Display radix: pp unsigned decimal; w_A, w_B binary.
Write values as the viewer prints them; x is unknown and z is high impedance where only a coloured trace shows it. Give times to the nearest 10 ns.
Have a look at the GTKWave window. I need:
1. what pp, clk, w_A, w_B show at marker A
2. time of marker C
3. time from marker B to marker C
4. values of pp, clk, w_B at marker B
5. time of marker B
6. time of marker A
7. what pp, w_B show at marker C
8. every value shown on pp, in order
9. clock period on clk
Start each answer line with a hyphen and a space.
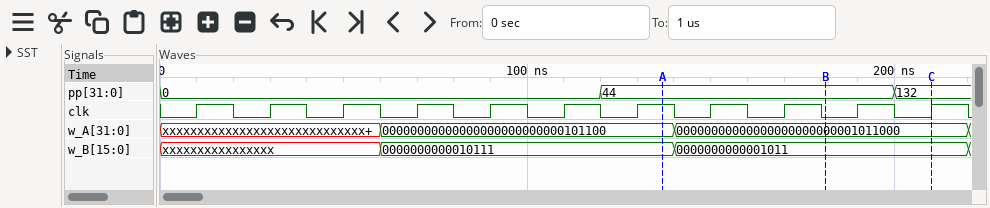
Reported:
- pp=44, clk=1, w_A=00000000000000000000000000101100, w_B=0000000000010111
- 210 ns
- 30 ns
- pp=44, clk=0, w_B=0000000000001011
- 180 ns
- 140 ns
- pp=132, w_B=0000000000001011
- 0, 44, 132
- 20 ns
